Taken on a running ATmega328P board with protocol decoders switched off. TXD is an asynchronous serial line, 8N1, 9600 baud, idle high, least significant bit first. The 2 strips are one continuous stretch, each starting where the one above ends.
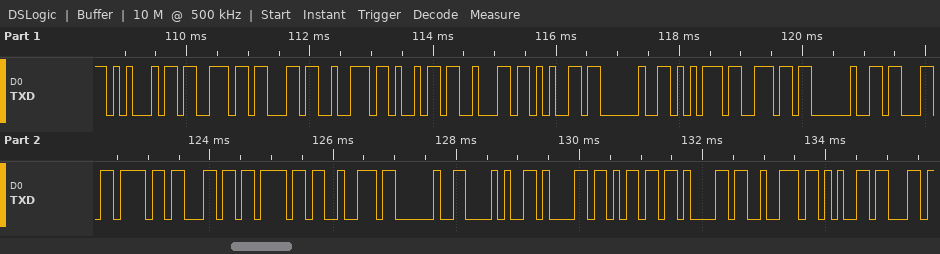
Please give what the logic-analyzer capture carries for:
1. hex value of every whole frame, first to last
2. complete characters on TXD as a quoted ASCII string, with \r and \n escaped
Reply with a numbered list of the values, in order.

1. 45 73 63 72 69 62 65 20 75 6E 20 63 6F 6C 6F 72 20 28 61 6D 61 72 65
2. "Escribe un color (amare"
